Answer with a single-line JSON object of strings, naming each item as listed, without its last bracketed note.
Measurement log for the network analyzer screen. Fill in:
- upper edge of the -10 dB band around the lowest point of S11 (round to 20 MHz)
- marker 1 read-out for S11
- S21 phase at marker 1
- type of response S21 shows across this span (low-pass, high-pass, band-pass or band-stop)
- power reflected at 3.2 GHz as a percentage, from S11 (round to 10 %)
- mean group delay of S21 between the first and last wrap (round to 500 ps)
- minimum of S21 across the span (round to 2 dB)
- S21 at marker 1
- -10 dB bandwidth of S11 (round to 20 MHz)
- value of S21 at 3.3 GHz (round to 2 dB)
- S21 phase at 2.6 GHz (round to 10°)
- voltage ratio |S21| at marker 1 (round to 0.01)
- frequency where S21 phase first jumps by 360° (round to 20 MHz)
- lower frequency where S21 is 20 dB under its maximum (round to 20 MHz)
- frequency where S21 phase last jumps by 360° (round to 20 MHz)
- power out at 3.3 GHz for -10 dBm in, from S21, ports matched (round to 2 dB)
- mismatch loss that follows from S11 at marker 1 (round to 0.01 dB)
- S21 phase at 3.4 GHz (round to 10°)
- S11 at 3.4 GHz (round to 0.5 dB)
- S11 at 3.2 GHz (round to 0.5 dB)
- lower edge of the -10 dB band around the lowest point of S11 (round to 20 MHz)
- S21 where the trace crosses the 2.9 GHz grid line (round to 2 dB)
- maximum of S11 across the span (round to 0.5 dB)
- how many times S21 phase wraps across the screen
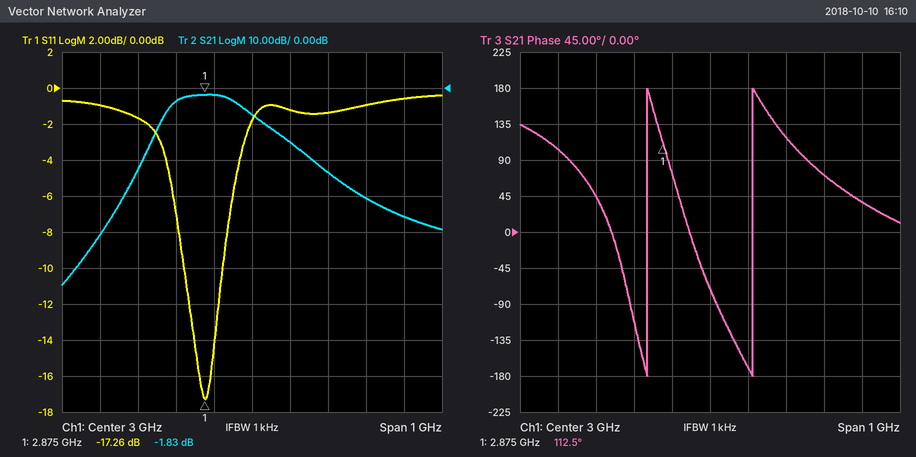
{"upper edge of the -10 dB band around the lowest point of S11": "2.92 GHz", "marker 1 read-out for S11": "-17.26 dB", "S21 phase at marker 1": "112.5°", "type of response S21 shows across this span": "band-pass", "power reflected at 3.2 GHz as a percentage, from S11": "70 %", "mean group delay of S21 between the first and last wrap": "3.5 ns", "minimum of S21 across the span": "-54 dB", "S21 at marker 1": "-1.83 dB", "-10 dB bandwidth of S11": "100 MHz", "value of S21 at 3.3 GHz": "-30 dB", "S21 phase at 2.6 GHz": "100°", "voltage ratio |S21| at marker 1": "0.81", "frequency where S21 phase first jumps by 360°": "2.84 GHz", "lower frequency where S21 is 20 dB under its maximum": "2.70 GHz", "frequency where S21 phase last jumps by 360°": "3.12 GHz", "power out at 3.3 GHz for -10 dBm in, from S21, ports matched": "-40 dBm", "mismatch loss that follows from S11 at marker 1": "0.08 dB", "S21 phase at 3.4 GHz": "40°", "S11 at 3.4 GHz": "-0.5 dB", "S11 at 3.2 GHz": "-1.5 dB", "lower edge of the -10 dB band around the lowest point of S11": "2.82 GHz", "S21 where the trace crosses the 2.9 GHz grid line": "-2 dB", "maximum of S11 across the span": "-0.5 dB", "how many times S21 phase wraps across the screen": "2"}
